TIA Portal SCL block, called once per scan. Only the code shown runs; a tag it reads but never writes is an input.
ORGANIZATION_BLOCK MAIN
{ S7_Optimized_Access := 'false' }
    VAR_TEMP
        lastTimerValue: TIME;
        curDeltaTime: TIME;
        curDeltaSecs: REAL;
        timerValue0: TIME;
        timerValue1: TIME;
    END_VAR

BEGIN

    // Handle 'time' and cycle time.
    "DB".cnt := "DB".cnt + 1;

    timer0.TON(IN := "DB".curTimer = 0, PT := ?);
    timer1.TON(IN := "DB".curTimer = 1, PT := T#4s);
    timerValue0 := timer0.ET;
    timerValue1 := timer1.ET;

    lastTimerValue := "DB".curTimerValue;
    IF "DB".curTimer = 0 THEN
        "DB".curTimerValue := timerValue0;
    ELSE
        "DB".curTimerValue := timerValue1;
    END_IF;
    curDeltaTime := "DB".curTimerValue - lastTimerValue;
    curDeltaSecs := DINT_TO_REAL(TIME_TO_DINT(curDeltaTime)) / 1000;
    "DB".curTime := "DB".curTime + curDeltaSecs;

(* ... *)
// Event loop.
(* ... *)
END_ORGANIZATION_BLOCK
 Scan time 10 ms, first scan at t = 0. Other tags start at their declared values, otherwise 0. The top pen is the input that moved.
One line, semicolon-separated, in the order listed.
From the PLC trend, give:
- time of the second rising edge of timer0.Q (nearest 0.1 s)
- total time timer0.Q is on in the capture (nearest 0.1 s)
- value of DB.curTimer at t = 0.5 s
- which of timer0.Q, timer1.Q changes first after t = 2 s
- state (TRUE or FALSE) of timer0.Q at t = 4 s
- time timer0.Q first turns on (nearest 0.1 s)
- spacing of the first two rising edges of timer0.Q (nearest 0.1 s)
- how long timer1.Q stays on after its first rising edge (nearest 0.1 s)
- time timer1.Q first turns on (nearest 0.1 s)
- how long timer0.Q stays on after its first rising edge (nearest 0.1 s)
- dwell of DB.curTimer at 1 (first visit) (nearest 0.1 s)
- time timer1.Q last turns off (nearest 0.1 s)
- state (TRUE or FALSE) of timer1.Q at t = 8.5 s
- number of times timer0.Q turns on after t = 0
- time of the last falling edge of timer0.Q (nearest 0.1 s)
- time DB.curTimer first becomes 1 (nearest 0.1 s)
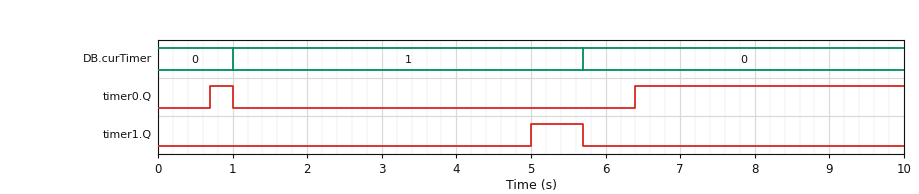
6.4 s; 3.9 s; 0; timer1.Q; FALSE; 0.7 s; 5.7 s; 0.7 s; 5.0 s; 0.3 s; 4.7 s; 5.7 s; FALSE; 2; 1.0 s; 1.0 s
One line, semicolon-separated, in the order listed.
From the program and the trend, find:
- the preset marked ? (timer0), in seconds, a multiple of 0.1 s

0.7 s
